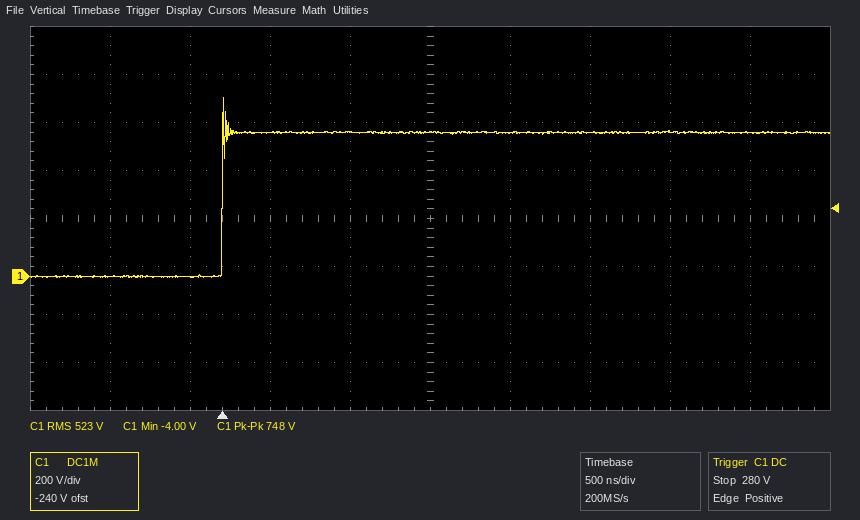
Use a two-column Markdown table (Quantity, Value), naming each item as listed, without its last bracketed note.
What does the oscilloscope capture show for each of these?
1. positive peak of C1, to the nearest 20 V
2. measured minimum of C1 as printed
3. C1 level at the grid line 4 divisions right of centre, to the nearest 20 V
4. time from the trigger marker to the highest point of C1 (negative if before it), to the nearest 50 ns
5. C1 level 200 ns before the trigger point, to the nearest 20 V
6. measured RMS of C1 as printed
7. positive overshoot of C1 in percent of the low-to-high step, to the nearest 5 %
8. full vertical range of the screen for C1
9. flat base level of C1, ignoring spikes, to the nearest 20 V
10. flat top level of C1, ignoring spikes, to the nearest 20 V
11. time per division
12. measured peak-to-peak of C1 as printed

| Quantity | Value |
|---|---|
| positive peak of C1, to the nearest 20 V | 740 V |
| measured minimum of C1 as printed | -4.00 V |
| C1 level at the grid line 4 divisions right of centre, to the nearest 20 V | 600 V |
| time from the trigger marker to the highest point of C1 (negative if before it), to the nearest 50 ns | 0 ns |
| C1 level 200 ns before the trigger point, to the nearest 20 V | 0 V |
| measured RMS of C1 as printed | 523 V |
| positive overshoot of C1 in percent of the low-to-high step, to the nearest 5 % | 25 % |
| full vertical range of the screen for C1 | 1.6 kV |
| flat base level of C1, ignoring spikes, to the nearest 20 V | 0 V |
| flat top level of C1, ignoring spikes, to the nearest 20 V | 600 V |
| time per division | 500 ns |
| measured peak-to-peak of C1 as printed | 748 V |
